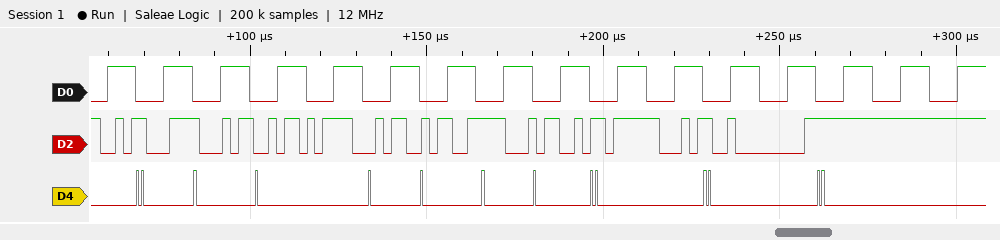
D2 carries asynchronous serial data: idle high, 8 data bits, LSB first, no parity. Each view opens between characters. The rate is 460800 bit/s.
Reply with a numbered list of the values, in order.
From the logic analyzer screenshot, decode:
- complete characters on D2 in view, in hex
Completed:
1. 1A, 34, EB, 34, F3, 34, FB, 34, 00
